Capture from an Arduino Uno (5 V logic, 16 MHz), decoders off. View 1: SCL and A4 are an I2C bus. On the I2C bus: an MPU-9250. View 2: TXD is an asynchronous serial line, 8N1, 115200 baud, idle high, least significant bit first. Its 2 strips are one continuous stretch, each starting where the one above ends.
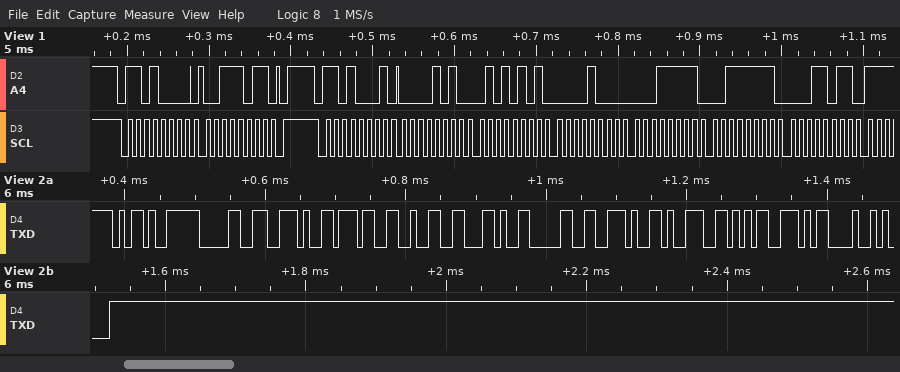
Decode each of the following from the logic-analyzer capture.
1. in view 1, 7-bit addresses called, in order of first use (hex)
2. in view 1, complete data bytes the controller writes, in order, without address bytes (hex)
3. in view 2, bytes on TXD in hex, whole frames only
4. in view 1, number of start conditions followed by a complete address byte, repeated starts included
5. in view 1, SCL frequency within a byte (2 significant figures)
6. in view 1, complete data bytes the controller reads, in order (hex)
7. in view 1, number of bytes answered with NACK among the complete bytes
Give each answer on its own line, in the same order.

0x68
3B
2D 30 2E 37 32 2C 30 2E 39 35 0D 0A
2
100 kHz
0A 55 08 1F 3F 1B
0
